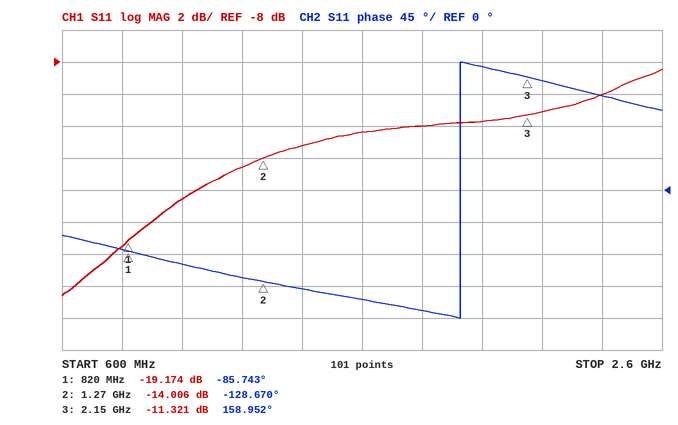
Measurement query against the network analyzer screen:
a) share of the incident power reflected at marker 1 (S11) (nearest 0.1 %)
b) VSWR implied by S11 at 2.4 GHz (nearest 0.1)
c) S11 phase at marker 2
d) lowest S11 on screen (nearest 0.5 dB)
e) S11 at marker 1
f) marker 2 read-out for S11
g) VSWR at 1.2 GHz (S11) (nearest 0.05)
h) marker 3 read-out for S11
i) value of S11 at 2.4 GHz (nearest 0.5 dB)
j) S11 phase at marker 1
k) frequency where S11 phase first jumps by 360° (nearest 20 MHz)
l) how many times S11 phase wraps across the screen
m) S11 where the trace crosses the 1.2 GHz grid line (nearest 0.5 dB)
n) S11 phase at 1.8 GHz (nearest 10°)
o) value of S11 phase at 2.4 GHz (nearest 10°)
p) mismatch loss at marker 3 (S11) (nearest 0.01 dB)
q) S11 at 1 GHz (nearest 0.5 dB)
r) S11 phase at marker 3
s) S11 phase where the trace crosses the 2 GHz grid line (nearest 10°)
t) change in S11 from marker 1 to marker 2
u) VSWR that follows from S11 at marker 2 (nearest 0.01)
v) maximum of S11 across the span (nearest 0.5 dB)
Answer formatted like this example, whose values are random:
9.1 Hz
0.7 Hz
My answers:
1.2 %
1.9
-128.670°
-22.5 dB
-19.174 dB
-14.006 dB
1.45
-11.321 dB
-10.0 dB
-85.743°
1.92 GHz
1
-14.5 dB
-170°
130°
0.33 dB
-16.5 dB
158.952°
170°
5.168 dB
1.50
-8.5 dB
